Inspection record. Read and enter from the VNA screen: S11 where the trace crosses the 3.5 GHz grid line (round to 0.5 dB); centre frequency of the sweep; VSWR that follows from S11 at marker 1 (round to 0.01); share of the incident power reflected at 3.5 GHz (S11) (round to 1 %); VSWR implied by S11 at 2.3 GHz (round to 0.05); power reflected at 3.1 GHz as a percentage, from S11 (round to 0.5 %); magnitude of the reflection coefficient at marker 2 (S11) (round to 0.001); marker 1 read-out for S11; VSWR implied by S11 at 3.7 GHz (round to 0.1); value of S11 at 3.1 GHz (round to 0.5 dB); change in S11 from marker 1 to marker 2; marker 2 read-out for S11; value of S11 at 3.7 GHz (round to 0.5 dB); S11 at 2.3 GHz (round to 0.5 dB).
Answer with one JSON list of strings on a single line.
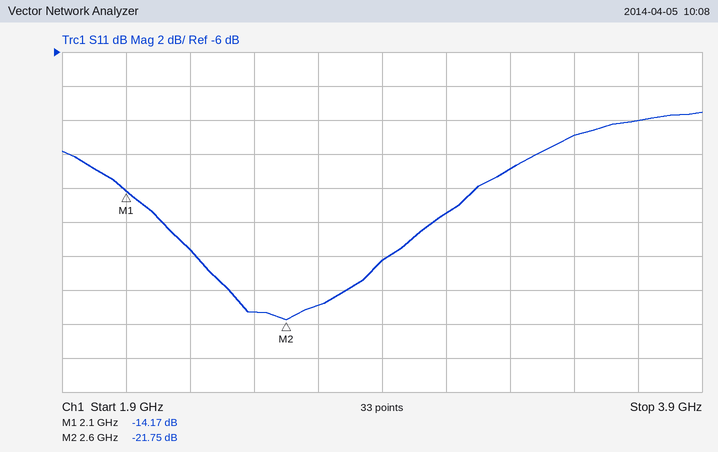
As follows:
["-11.0 dB", "2.9 GHz", "1.49", "8 %", "1.30", "3.0 %", "0.082", "-14.17 dB", "1.9", "-15.5 dB", "-7.58 dB", "-21.75 dB", "-10.0 dB", "-17.5 dB"]
